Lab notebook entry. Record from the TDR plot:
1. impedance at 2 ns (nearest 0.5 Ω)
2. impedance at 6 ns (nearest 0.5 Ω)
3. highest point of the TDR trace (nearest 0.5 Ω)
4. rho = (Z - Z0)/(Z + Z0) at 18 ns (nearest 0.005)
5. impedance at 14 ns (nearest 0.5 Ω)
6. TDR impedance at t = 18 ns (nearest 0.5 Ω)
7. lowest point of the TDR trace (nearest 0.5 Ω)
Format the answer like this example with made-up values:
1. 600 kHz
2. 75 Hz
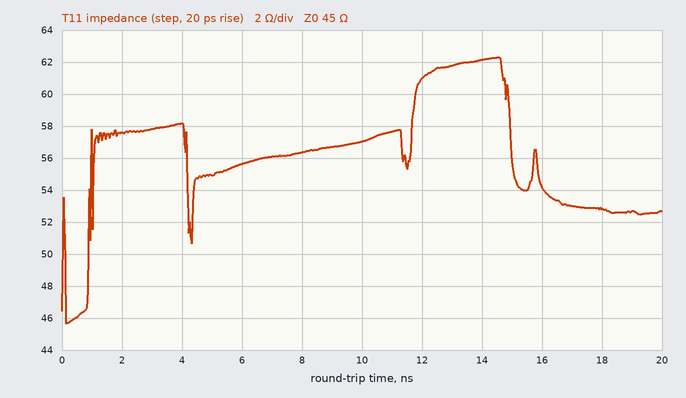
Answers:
1. 57.5 Ω
2. 55.5 Ω
3. 62.5 Ω
4. +0.080
5. 62.0 Ω
6. 53.0 Ω
7. 45.5 Ω
